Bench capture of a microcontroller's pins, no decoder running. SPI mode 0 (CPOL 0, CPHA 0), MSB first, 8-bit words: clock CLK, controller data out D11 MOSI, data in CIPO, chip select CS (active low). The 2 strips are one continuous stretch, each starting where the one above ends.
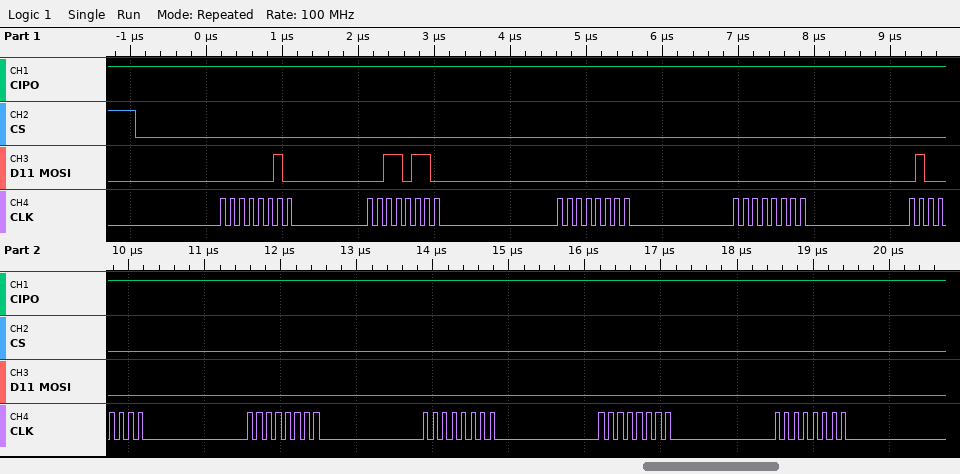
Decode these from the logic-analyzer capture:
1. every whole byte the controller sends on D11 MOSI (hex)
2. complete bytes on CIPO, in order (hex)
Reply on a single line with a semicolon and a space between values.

0x02 0x36 0x00 0x00 0x40 0x00 0x00 0x00 0x00; 0xFF 0xFF 0xFF 0xFF 0xFF 0xFF 0xFF 0xFF 0xFF
